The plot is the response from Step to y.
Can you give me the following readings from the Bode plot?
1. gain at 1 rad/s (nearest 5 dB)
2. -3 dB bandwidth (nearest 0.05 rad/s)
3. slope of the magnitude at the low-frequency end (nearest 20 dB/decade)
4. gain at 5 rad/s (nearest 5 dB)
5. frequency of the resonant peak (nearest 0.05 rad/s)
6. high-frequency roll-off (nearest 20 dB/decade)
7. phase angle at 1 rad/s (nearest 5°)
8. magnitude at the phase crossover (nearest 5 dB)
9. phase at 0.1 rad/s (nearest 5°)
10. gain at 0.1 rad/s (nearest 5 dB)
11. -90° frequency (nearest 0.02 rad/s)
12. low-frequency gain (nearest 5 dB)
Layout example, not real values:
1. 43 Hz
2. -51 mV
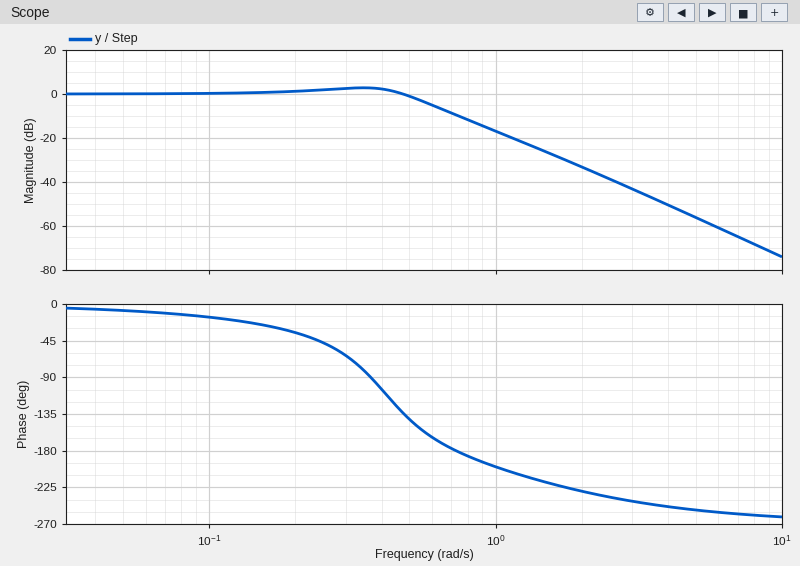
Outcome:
1. -15 dB
2. 0.55 rad/s
3. 0 dB/decade
4. -55 dB
5. 0.35 rad/s
6. -60 dB/decade
7. -200°
8. -10 dB
9. -15°
10. 0 dB
11. 0.36 rad/s
12. 0 dB
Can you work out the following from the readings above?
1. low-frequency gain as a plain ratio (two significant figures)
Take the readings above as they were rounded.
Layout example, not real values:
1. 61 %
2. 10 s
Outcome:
1. 1.0
